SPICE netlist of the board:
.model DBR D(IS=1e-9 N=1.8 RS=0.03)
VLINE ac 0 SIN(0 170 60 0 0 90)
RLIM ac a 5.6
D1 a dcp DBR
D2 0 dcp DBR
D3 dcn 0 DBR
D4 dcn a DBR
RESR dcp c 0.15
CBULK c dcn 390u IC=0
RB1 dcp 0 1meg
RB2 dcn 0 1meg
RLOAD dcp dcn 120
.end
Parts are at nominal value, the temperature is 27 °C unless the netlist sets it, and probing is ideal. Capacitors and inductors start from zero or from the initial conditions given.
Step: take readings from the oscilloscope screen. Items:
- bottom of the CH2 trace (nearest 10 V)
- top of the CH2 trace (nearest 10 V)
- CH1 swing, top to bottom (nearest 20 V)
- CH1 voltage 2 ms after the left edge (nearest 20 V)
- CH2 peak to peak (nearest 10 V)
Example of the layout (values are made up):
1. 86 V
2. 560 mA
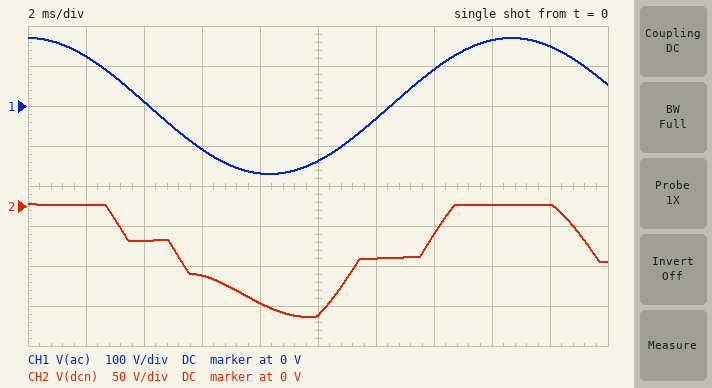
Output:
1. -140 V
2. 0 V
3. 340 V
4. 120 V
5. 140 V
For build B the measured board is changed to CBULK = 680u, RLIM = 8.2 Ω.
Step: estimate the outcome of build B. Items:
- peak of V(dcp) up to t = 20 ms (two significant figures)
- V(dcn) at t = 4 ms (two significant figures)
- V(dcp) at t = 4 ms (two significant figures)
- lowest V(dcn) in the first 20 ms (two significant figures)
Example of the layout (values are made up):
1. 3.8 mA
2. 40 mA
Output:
1. 120 V
2. -26 V
3. 26 V
4. -100 V
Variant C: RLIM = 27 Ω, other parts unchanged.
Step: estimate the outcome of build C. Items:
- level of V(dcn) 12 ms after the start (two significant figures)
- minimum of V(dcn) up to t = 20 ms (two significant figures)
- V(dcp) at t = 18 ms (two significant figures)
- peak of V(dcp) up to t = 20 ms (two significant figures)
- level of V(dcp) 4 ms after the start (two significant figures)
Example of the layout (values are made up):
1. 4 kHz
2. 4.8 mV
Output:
1. -35 V
2. -72 V
3. 89 V
4. 90 V
5. 16 V
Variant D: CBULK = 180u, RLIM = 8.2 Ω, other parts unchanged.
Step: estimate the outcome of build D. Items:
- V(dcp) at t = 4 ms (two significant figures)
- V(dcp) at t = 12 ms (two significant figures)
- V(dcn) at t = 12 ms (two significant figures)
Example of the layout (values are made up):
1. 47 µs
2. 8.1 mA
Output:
1. 48 V
2. 64 V
3. -64 V
